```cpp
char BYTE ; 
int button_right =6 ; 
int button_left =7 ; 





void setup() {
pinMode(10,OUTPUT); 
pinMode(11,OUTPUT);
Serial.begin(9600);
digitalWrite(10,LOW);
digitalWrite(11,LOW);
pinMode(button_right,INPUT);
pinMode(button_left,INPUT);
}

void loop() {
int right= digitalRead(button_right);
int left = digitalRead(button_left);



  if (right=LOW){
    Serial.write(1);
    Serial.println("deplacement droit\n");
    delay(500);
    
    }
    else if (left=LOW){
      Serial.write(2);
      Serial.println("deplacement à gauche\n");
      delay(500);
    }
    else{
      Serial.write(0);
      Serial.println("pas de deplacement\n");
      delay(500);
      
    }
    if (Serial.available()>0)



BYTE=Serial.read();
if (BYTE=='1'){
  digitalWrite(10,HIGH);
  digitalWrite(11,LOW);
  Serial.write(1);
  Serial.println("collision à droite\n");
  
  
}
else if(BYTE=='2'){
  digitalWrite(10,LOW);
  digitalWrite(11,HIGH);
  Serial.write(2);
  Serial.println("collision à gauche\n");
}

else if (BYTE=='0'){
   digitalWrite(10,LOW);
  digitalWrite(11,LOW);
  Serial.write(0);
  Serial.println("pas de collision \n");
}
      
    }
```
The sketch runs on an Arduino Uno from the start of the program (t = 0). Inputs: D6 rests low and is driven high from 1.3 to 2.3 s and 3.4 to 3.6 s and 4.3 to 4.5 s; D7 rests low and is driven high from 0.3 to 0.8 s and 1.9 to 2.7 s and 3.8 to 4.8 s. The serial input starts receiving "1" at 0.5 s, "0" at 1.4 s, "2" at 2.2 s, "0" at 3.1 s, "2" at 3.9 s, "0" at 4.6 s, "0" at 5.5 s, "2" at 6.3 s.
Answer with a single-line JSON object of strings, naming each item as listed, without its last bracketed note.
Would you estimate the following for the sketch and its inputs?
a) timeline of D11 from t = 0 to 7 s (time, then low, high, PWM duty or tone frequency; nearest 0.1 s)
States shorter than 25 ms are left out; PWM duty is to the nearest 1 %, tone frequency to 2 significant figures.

{"timeline of D11 from t = 0 to 7 s": "0 s low; 2.5 s high; 3.5 s low; 4 s high; 5 s low; 6.5 s high"}
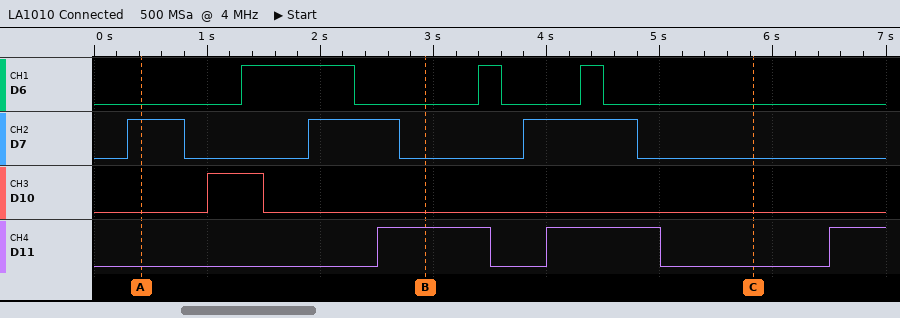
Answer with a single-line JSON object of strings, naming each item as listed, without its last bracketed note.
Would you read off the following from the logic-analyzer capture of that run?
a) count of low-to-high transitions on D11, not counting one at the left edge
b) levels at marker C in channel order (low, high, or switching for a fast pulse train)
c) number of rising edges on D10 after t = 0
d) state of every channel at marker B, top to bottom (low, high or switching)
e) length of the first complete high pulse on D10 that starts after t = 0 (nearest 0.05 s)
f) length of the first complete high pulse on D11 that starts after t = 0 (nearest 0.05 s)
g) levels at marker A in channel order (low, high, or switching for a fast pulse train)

{"count of low-to-high transitions on D11, not counting one at the left edge": "3", "levels at marker C in channel order": "D6 low, D7 low, D10 low, D11 low", "number of rising edges on D10 after t = 0": "1", "state of every channel at marker B, top to bottom": "D6 low, D7 low, D10 low, D11 high", "length of the first complete high pulse on D10 that starts after t = 0": "0.50 s", "length of the first complete high pulse on D11 that starts after t = 0": "1.00 s", "levels at marker A in channel order": "D6 low, D7 high, D10 low, D11 low"}
